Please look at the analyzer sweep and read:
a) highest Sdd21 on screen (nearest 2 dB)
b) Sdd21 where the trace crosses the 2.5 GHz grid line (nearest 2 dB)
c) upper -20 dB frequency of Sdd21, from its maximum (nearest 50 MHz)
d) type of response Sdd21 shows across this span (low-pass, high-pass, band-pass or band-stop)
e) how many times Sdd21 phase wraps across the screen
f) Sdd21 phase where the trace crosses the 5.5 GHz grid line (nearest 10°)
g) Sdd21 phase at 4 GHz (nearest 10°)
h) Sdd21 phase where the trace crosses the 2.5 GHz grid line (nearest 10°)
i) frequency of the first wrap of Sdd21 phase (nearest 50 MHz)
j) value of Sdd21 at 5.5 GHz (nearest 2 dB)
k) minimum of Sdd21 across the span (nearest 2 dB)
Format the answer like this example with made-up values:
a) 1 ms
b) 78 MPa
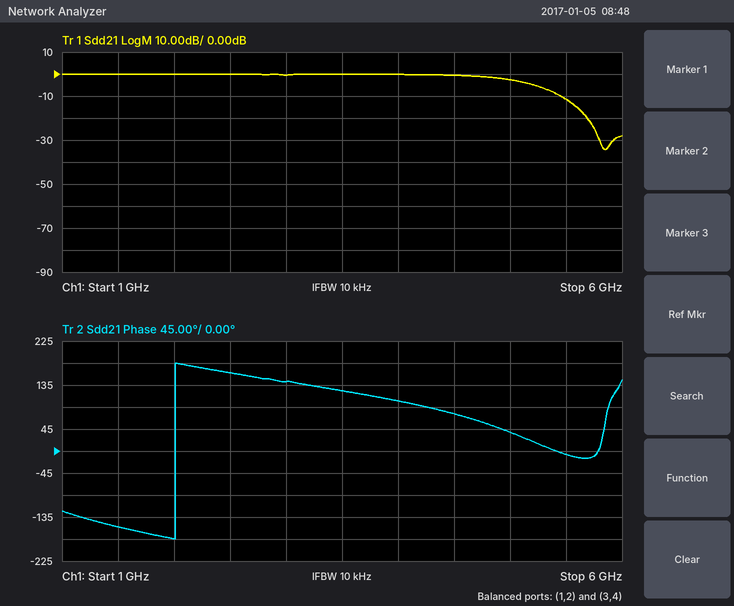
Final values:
a) 0 dB
b) 0 dB
c) 5.70 GHz
d) low-pass
e) 1
f) -10°
g) 100°
h) 160°
i) 2.00 GHz
j) -12 dB
k) -34 dB
